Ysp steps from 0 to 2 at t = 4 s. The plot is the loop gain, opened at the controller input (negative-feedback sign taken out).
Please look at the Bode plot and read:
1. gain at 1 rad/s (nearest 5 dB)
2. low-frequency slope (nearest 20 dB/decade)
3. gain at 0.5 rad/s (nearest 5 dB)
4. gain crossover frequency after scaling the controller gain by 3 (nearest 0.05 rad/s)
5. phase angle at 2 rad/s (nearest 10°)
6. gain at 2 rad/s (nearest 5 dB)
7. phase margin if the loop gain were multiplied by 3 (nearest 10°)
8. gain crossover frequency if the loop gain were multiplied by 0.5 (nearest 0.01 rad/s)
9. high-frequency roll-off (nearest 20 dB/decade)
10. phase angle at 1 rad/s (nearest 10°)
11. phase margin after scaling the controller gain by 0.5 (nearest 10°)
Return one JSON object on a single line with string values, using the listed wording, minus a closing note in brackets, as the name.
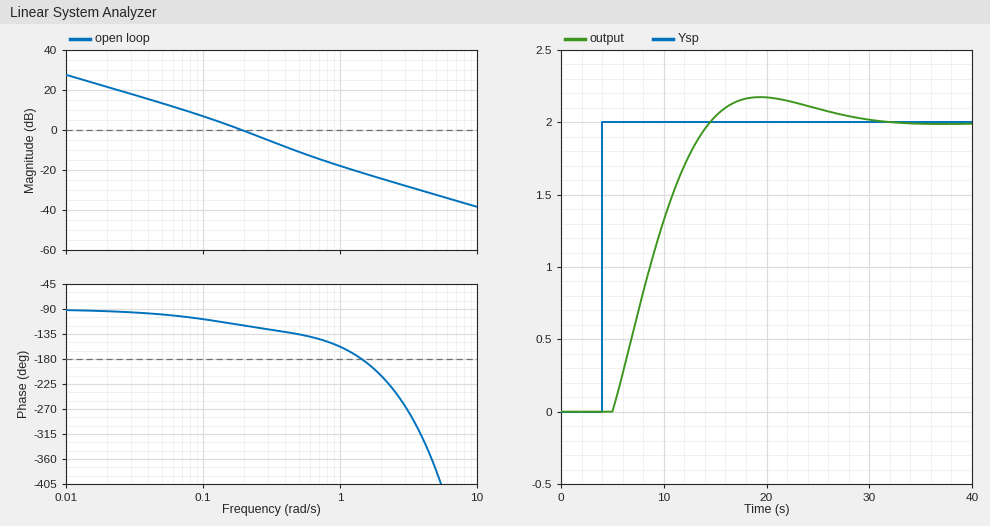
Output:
{"gain at 1 rad/s": "-20 dB", "low-frequency slope": "-20 dB/decade", "gain at 0.5 rad/s": "-10 dB", "gain crossover frequency after scaling the controller gain by 3": "0.45 rad/s", "phase angle at 2 rad/s": "-210°", "gain at 2 rad/s": "-25 dB", "phase margin if the loop gain were multiplied by 3": "50°", "gain crossover frequency if the loop gain were multiplied by 0.5": "0.11 rad/s", "high-frequency roll-off": "-20 dB/decade", "phase angle at 1 rad/s": "-160°", "phase margin after scaling the controller gain by 0.5": "70°"}
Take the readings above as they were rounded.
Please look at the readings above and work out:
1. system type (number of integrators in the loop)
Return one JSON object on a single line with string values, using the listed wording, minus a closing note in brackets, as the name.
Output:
{"system type": "1"}
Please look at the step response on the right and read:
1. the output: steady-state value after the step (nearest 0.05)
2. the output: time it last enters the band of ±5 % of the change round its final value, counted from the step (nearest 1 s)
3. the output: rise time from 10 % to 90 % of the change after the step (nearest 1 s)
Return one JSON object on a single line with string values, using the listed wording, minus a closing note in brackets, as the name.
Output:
{"the output: steady-state value after the step": "2.00", "the output: time it last enters the band of ±5 % of the change round its final value, counted from the step": "21 s", "the output: rise time from 10 % to 90 % of the change after the step": "7 s"}
